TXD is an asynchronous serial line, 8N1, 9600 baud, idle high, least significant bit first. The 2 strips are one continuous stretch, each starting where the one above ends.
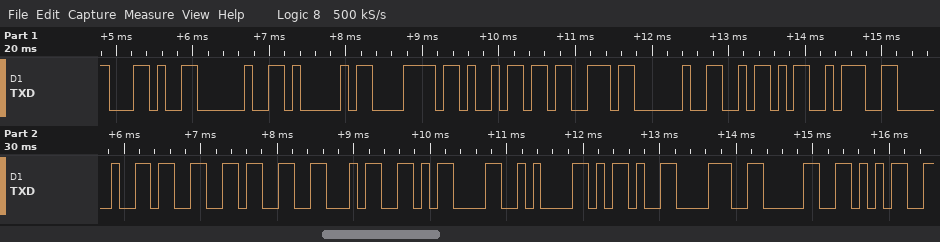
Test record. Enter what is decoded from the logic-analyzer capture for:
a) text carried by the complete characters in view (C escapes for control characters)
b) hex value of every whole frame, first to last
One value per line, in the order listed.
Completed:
", Axis Z: 334\r\n-805"
0x2C 0x20 0x41 0x78 0x69 0x73 0x20 0x5A 0x3A 0x20 0x33 0x33 0x34 0x0D 0x0A 0x2D 0x38 0x30 0x35
